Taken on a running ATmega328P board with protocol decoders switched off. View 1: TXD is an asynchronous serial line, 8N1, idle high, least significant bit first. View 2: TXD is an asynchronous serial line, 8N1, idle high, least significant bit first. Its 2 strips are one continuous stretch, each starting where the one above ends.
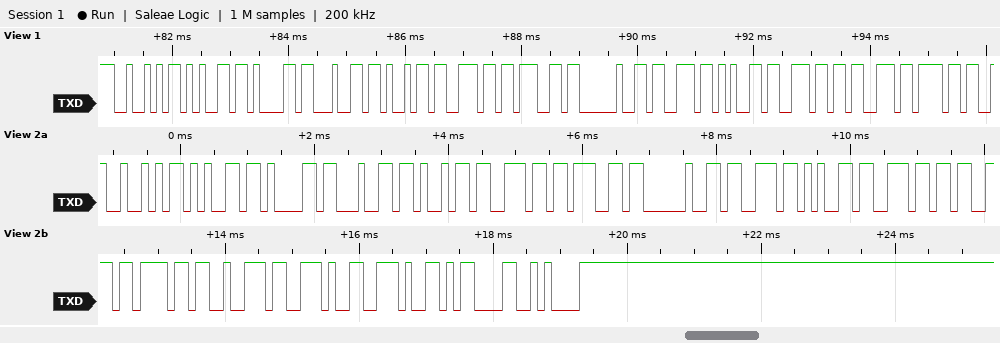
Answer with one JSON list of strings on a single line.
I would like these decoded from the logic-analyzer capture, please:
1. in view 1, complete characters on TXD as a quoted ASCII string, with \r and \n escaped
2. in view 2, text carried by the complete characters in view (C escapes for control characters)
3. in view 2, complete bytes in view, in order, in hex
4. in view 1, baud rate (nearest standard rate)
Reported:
["\"Reading senso\"", "\"Reading sensor..\\r\\n\"", "52 65 61 64 69 6E 67 20 73 65 6E 73 6F 72 2E 2E 0D 0A", "9600 baud"]
